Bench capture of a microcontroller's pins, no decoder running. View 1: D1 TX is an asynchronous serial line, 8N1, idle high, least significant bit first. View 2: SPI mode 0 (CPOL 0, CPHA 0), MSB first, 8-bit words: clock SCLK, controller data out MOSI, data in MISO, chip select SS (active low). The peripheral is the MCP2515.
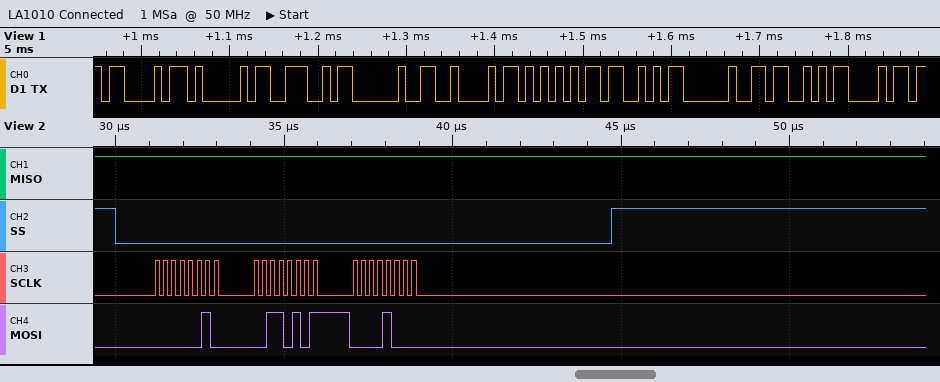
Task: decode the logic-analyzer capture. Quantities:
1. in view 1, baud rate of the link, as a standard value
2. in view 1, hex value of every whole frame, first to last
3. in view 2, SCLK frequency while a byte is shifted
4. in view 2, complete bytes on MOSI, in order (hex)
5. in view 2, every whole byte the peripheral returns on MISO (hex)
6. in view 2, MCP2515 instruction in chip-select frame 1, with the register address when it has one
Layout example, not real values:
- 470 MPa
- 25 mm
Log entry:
- 115200 baud
- 0x43 0x41 0x4E 0x20 0x42 0x55 0x53 0x20 0x53 0x68
- 4 MHz
- 0x02 0x35 0x08
- 0xFF 0xFF 0xFF
- WRITE 0x35
